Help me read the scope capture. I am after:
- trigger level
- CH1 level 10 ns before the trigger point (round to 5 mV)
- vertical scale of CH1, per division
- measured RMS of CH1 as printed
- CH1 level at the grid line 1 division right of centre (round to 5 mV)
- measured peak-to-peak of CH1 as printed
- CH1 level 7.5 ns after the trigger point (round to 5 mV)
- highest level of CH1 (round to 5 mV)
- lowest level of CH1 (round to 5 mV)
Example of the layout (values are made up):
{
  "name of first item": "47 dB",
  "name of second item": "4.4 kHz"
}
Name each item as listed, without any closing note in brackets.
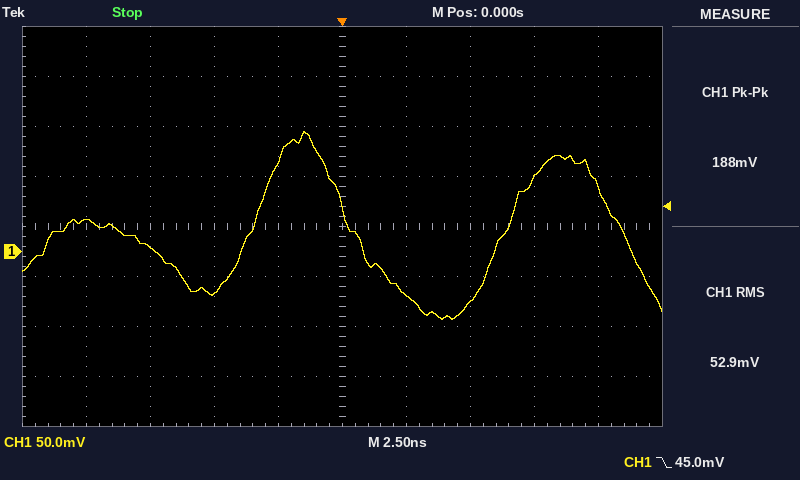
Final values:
{
  "trigger level": "45.0 mV",
  "CH1 level 10 ns before the trigger point": "30 mV",
  "vertical scale of CH1, per division": "50 mV",
  "measured RMS of CH1 as printed": "52.9 mV",
  "CH1 level at the grid line 1 division right of centre": "-45 mV",
  "measured peak-to-peak of CH1 as printed": "188 mV",
  "CH1 level 7.5 ns after the trigger point": "75 mV",
  "highest level of CH1": "120 mV",
  "lowest level of CH1": "-70 mV"
}
